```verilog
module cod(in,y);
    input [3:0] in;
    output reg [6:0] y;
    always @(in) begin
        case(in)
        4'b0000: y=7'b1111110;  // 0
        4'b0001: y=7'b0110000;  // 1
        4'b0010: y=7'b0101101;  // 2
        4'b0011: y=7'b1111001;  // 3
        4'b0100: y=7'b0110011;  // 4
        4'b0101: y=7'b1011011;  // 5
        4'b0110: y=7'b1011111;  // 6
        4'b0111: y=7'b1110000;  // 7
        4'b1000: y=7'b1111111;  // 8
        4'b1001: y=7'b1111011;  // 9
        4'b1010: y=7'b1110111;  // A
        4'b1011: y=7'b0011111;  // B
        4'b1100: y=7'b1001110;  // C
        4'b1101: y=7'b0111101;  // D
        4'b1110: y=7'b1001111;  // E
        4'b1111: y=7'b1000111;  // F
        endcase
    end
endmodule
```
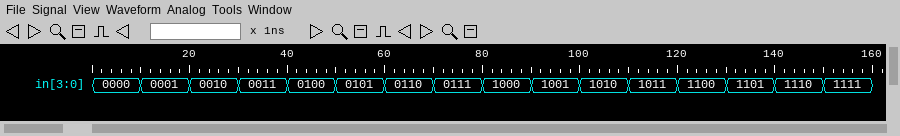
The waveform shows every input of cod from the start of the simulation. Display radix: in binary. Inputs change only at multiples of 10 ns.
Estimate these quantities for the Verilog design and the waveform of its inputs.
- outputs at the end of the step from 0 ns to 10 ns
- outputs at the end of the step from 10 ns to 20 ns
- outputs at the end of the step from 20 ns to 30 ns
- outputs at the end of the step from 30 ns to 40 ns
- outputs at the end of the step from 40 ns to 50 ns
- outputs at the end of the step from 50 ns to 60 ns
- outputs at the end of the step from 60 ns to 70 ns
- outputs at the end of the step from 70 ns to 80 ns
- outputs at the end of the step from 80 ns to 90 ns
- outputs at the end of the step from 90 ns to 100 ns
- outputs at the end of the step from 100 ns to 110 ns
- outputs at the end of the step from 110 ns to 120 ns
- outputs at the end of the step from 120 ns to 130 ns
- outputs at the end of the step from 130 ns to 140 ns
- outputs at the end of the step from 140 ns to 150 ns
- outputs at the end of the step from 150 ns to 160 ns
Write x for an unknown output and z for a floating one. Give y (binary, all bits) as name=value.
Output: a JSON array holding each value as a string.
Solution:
["y=1111110", "y=0110000", "y=0101101", "y=1111001", "y=0110011", "y=1011011", "y=1011111", "y=1110000", "y=1111111", "y=1111011", "y=1110111", "y=0011111", "y=1001110", "y=0111101", "y=1001111", "y=1000111"]
